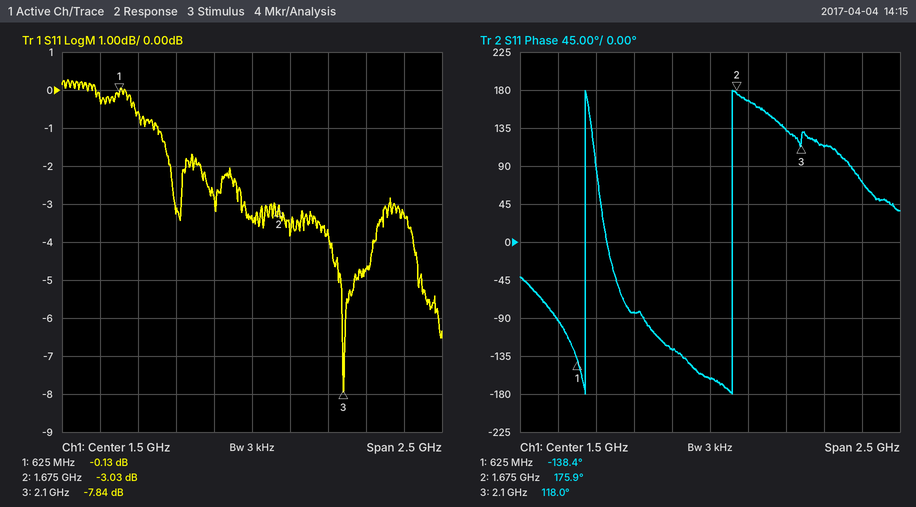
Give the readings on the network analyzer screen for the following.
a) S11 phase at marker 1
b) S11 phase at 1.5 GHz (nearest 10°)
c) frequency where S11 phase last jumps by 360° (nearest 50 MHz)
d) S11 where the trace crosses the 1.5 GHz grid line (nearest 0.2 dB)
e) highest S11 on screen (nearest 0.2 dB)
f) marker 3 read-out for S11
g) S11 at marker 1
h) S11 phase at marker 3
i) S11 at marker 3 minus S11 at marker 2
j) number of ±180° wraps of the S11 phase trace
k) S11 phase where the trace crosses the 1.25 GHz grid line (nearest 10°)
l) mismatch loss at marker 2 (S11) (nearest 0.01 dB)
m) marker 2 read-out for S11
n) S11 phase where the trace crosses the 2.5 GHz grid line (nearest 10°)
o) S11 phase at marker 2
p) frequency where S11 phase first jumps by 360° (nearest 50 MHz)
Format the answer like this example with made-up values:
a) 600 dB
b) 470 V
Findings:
a) -138.4°
b) -160°
c) 1.65 GHz
d) -3.4 dB
e) 0.2 dB
f) -7.84 dB
g) -0.13 dB
h) 118.0°
i) -4.81 dB
j) 2
k) -130°
l) 2.99 dB
m) -3.03 dB
n) 70°
o) 175.9°
p) 700 MHz
